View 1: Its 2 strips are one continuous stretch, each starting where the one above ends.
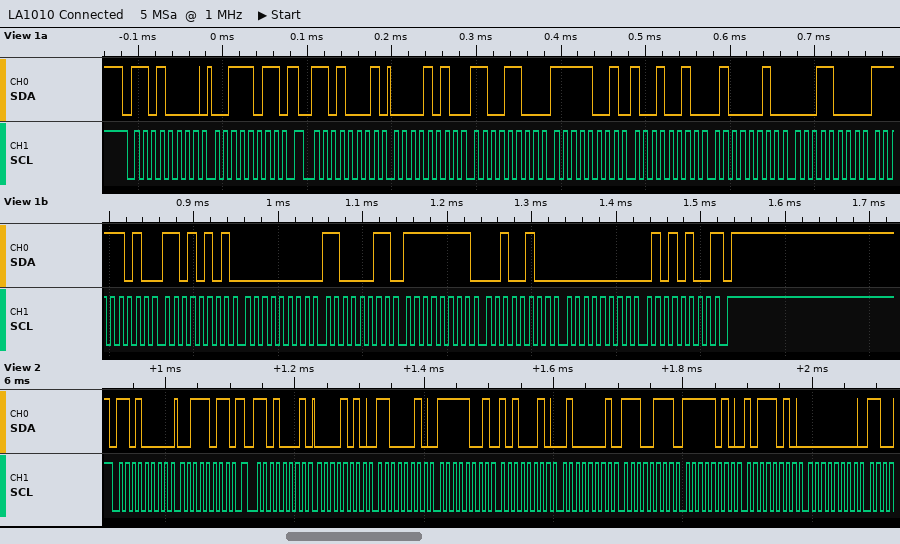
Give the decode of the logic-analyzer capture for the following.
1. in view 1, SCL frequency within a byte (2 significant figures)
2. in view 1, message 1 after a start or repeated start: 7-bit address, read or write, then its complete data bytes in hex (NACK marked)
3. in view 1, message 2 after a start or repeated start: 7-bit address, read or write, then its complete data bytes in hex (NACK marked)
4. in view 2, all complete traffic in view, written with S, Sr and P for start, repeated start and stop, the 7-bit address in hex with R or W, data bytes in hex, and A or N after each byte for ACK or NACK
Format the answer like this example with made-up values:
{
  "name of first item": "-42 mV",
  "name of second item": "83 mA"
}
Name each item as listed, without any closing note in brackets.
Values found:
{
  "in view 1, SCL frequency within a byte": "100 kHz",
  "in view 1, message 1 after a start or repeated start: 7-bit address, read or write, then its complete data bytes in hex": "0x68 write: 3B",
  "in view 1, message 2 after a start or repeated start: 7-bit address, read or write, then its complete data bytes in hex": "0x68 read: 0A CC F9 92 42 18 FA D5 00 C3 FF 24 00 54 NACK",
  "in view 2, all complete traffic in view, written with S, Sr and P for start, repeated start and stop, the 7-bit address in hex with R or W, data bytes in hex, and A or N after each byte for ACK or NACK": "S 68W A 3B A Sr 68R A 0A A C2 A F9 A A2 A 41 A E7 A FA A BA A 00 A"
}
